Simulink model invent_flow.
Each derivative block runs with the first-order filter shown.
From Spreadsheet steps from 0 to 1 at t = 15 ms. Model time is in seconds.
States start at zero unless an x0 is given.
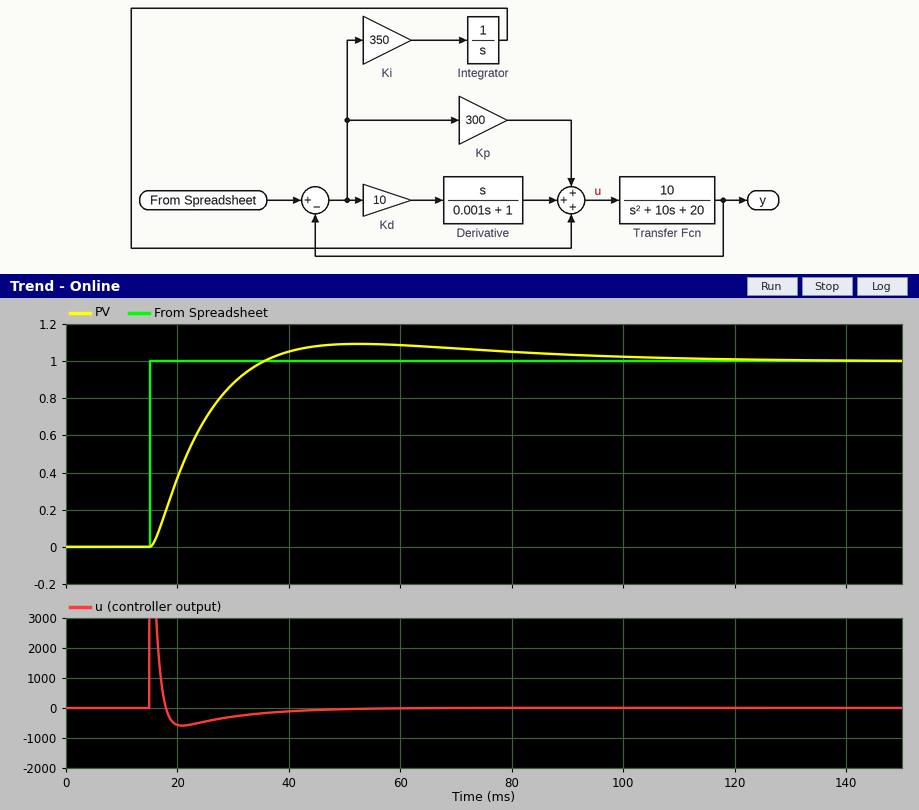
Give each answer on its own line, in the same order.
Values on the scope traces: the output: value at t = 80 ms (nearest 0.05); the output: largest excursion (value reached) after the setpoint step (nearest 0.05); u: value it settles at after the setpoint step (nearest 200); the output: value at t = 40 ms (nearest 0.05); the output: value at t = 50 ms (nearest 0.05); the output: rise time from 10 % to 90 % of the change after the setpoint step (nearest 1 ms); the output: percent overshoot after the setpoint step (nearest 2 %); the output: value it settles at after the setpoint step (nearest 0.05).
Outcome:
1.05
1.10
0
1.05
1.10
14 ms
10 %
1.00
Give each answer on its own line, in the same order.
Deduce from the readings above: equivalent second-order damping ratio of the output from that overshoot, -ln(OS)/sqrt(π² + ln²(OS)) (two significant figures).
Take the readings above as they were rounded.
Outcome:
0.59
